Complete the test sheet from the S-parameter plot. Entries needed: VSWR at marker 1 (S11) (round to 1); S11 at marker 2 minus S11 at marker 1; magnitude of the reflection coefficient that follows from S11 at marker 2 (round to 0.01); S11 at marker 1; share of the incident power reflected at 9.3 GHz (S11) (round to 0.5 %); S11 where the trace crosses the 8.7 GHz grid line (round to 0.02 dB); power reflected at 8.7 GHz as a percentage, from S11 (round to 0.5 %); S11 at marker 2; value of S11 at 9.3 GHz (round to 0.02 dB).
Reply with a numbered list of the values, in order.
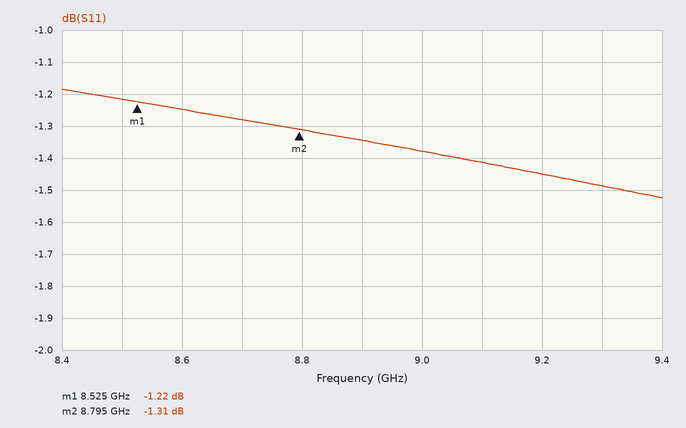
1. 14
2. -0.09 dB
3. 0.86
4. -1.22 dB
5. 71.0 %
6. -1.28 dB
7. 74.5 %
8. -1.31 dB
9. -1.48 dB
